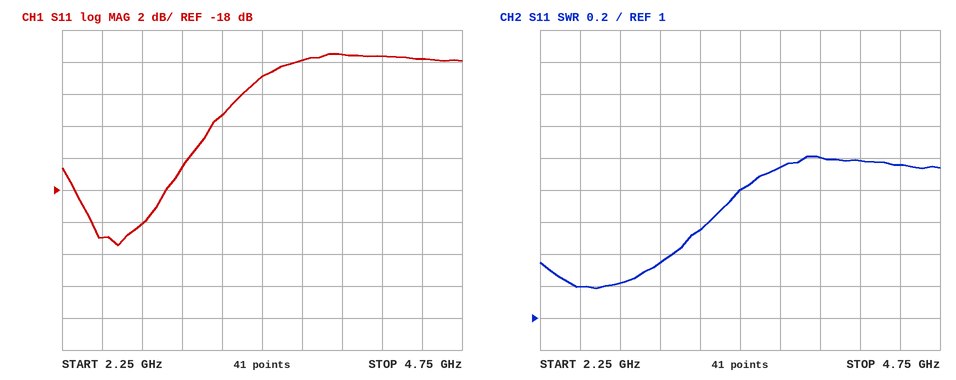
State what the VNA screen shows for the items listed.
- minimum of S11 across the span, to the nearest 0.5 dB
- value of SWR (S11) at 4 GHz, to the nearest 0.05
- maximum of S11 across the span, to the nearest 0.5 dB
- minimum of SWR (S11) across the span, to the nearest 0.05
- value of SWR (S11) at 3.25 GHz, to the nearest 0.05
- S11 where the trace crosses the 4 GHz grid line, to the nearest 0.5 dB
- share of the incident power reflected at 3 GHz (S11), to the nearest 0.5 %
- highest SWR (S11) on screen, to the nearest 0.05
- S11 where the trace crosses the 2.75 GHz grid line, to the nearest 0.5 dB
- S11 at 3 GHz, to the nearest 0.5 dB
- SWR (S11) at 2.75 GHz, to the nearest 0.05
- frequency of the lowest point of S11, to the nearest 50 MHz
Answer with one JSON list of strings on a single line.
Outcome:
["-21.5 dB", "2.00", "-9.5 dB", "1.20", "1.55", "-9.5 dB", "2.0 %", "2.00", "-20.0 dB", "-16.5 dB", "1.20", "2.60 GHz"]
